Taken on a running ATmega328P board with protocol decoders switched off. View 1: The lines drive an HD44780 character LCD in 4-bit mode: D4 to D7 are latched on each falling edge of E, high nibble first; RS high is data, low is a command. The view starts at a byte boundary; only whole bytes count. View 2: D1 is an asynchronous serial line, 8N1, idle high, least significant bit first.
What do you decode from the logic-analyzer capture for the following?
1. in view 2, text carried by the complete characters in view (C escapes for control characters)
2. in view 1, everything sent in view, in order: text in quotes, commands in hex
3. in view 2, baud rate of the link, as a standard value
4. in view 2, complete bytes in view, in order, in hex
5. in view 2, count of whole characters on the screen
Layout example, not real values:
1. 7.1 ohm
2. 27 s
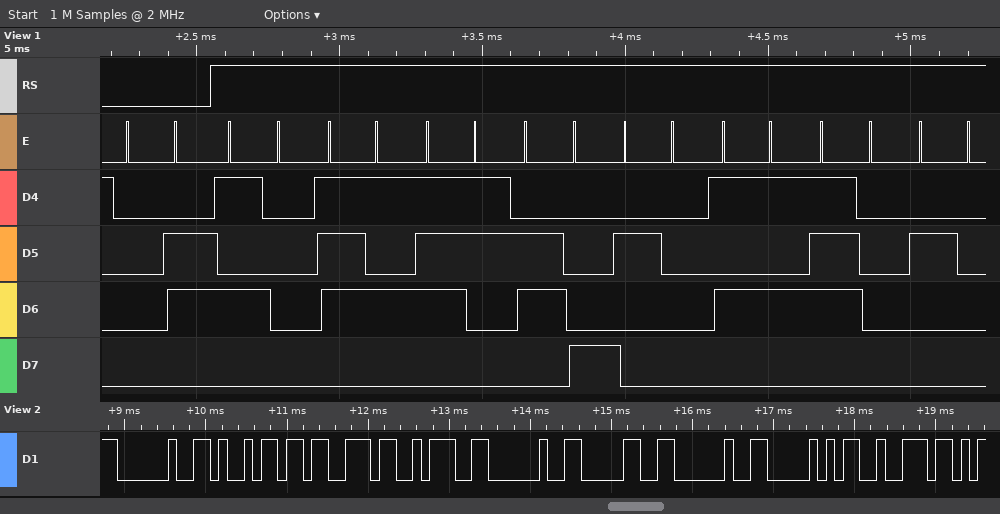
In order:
1. " is: 0 Pr"
2. 0x06 "Push Up "
3. 9600 baud
4. 20 69 73 3A 20 30 20 50 72
5. 9
